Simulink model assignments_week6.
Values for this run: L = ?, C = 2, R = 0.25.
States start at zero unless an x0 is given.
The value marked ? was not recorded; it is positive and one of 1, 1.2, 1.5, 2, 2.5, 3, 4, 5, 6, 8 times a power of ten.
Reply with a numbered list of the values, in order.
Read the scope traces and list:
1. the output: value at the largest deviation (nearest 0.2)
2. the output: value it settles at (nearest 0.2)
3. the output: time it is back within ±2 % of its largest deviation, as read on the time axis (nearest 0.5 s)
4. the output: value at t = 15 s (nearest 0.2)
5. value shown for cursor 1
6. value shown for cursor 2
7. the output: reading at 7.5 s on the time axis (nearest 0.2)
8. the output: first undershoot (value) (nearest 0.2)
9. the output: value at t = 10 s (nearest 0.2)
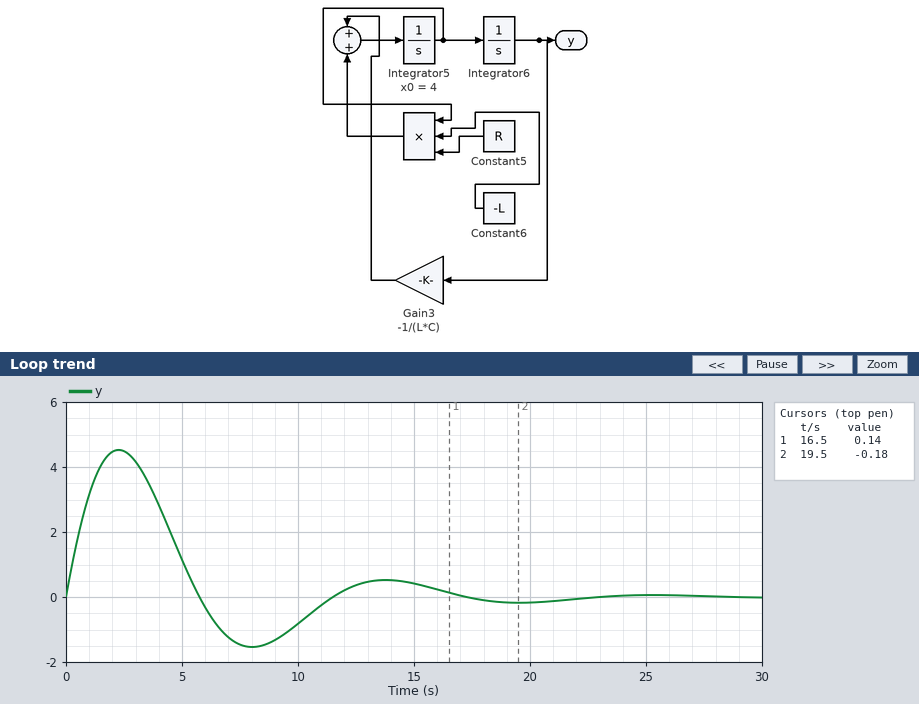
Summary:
1. 4.6
2. 0.0
3. 21.5 s
4. 0.4
5. 0.14
6. -0.18
7. -1.4
8. -1.6
9. -0.8
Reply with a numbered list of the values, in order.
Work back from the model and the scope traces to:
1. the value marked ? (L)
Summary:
1. 1.5
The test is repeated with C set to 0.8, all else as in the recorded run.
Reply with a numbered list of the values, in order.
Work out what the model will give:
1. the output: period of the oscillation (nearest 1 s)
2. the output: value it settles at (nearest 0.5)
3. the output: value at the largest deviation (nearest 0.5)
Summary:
1. 7 s
2. 0.0
3. 3.5
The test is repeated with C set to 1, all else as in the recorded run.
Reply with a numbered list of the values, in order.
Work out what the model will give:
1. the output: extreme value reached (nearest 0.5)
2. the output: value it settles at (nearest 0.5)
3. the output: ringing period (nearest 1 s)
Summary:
1. 3.5
2. 0.0
3. 8 s
